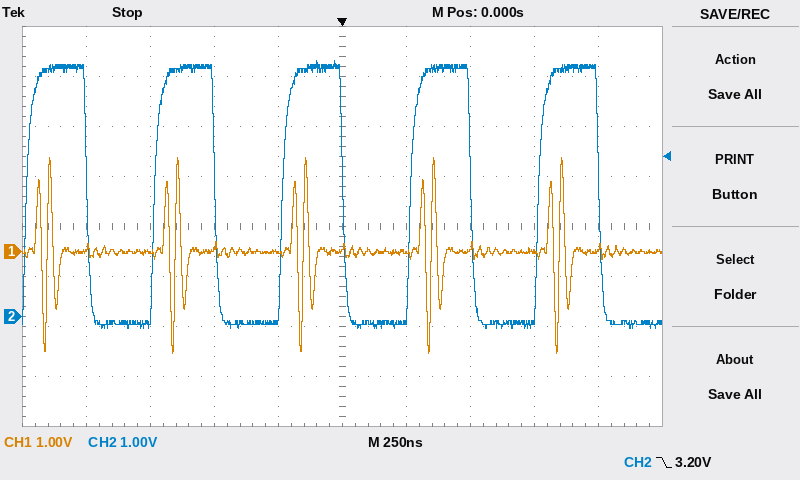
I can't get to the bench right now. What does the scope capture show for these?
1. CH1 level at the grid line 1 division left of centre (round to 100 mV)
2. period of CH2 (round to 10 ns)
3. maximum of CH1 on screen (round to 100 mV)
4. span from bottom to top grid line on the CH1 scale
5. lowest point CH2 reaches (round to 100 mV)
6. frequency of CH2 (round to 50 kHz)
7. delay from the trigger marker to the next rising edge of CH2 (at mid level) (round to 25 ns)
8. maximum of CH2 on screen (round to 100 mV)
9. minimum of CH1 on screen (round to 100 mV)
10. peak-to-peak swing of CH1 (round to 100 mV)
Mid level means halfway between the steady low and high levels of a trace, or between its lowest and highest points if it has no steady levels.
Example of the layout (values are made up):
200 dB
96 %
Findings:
0.0 V
500 ns
1.9 V
8 V
-200 mV
2.00 MHz
275 ns
5.1 V
-2.0 V
3.9 V
